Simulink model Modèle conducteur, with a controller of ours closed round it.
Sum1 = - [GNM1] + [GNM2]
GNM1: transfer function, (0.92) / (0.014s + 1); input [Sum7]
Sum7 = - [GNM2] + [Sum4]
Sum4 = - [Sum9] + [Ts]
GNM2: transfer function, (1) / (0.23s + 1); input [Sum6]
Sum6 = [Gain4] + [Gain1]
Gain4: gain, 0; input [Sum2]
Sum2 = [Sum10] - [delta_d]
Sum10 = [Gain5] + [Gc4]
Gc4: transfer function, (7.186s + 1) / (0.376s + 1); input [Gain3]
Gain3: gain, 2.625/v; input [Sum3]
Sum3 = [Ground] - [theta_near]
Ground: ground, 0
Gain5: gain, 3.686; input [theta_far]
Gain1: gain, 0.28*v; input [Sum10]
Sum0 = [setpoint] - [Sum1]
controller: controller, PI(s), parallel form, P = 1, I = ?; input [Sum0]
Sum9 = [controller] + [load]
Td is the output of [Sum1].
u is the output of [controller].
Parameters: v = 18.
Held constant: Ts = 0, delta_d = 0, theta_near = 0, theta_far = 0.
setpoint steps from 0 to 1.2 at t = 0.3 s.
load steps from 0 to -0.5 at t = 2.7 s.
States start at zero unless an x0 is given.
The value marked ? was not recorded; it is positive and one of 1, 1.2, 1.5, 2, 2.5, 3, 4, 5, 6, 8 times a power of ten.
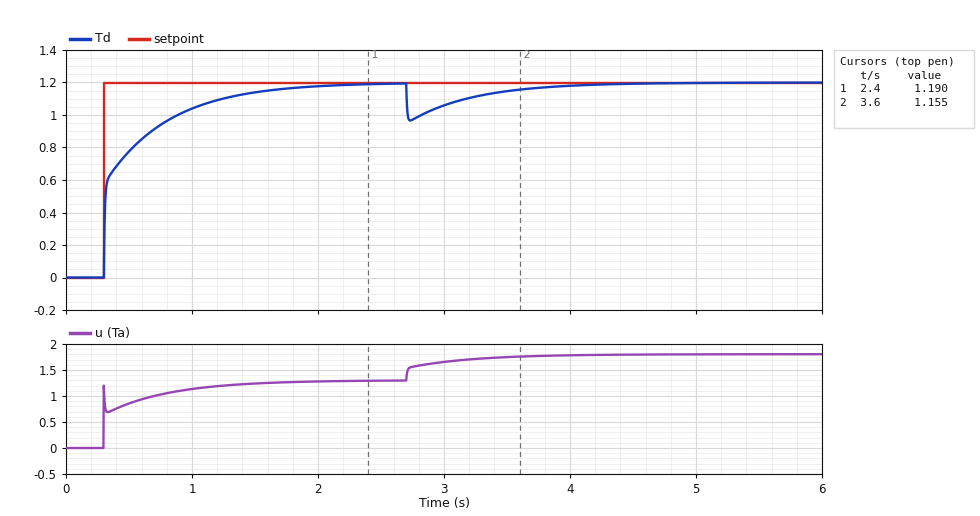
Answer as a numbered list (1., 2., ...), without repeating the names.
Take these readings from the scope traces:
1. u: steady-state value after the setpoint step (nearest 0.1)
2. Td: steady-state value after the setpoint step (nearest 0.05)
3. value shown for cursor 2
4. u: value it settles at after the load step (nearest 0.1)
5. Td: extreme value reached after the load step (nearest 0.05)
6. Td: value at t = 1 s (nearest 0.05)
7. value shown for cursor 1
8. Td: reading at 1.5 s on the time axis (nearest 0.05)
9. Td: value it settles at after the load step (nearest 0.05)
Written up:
1. 1.3
2. 1.20
3. 1.155
4. 1.8
5. 0.95
6. 1.05
7. 1.190
8. 1.15
9. 1.20
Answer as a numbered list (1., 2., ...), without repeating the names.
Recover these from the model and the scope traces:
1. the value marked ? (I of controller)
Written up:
1. 4
